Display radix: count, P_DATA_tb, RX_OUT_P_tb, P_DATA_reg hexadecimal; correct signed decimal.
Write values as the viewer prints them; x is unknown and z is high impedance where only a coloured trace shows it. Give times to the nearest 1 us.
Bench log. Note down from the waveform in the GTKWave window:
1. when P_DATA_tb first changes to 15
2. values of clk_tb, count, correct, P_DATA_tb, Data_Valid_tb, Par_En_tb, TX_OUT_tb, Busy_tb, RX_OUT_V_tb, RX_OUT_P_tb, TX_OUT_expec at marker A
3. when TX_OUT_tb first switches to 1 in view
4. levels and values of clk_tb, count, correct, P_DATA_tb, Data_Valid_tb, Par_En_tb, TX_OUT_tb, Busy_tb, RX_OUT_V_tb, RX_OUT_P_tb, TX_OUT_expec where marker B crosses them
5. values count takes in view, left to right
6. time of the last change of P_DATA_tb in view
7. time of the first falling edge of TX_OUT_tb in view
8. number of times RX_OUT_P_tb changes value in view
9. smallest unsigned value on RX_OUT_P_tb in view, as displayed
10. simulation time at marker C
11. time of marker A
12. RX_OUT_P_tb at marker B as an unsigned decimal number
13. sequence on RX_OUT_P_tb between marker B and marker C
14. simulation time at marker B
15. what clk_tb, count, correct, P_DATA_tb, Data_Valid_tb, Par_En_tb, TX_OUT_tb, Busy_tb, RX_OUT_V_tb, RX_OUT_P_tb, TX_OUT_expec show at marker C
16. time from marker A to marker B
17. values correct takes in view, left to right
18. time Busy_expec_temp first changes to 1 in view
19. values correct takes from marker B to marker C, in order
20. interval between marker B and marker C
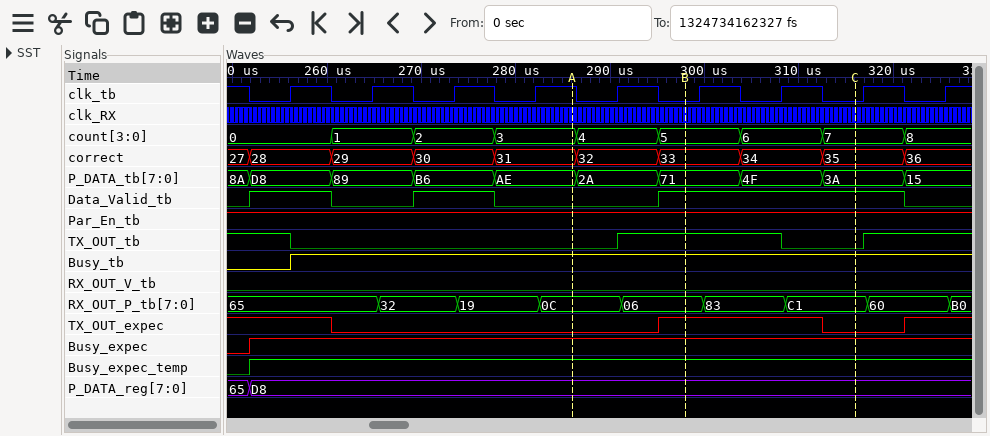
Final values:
321 us
clk_tb=1, count=3, correct=31, P_DATA_tb=AE, Data_Valid_tb=0, Par_En_tb=1, TX_OUT_tb=0, Busy_tb=1, RX_OUT_V_tb=0, RX_OUT_P_tb=0C, TX_OUT_expec=0
291 us
clk_tb=0, count=5, correct=33, P_DATA_tb=71, Data_Valid_tb=1, Par_En_tb=1, TX_OUT_tb=1, Busy_tb=1, RX_OUT_V_tb=0, RX_OUT_P_tb=06, TX_OUT_expec=1
0, 1, 2, 3, 4, 5, 6, 7, 8
321 us
256 us
8
06
316 us
286 us
6
06, 83, C1
298 us
clk_tb=0, count=7, correct=35, P_DATA_tb=3A, Data_Valid_tb=1, Par_En_tb=1, TX_OUT_tb=0, Busy_tb=1, RX_OUT_V_tb=0, RX_OUT_P_tb=C1, TX_OUT_expec=0
12 us
27, 28, 29, 30, 31, 32, 33, 34, 35, 36
252 us
33, 34, 35
18 us
